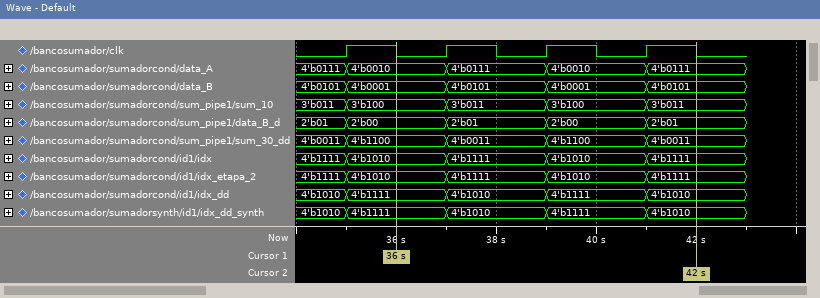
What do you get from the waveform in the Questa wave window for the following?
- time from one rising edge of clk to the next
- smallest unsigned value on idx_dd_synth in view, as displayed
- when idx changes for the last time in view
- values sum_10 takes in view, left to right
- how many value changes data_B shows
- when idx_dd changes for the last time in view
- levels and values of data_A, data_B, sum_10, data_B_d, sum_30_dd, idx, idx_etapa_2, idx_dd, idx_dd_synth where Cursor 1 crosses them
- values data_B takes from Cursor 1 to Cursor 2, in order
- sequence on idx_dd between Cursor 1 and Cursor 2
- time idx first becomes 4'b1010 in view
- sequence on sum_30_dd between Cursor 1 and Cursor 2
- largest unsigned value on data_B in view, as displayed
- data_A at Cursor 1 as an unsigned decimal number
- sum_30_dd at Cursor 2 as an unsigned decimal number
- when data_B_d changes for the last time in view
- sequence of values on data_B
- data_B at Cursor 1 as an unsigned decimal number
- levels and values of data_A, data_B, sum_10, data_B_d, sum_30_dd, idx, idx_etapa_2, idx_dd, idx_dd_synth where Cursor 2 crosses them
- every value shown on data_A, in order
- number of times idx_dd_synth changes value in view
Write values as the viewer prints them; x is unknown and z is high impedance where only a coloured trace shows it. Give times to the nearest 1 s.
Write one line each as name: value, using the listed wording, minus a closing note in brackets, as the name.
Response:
time from one rising edge of clk to the next: 2 s
smallest unsigned value on idx_dd_synth in view, as displayed: 4'b1010
when idx changes for the last time in view: 41 s
values sum_10 takes in view, left to right: 3'b011, 3'b100, 3'b011, 3'b100, 3'b011
how many value changes data_B shows: 4
when idx_dd changes for the last time in view: 41 s
levels and values of data_A, data_B, sum_10, data_B_d, sum_30_dd, idx, idx_etapa_2, idx_dd, idx_dd_synth where Cursor 1 crosses them: data_A=4'b0010, data_B=4'b0001, sum_10=3'b100, data_B_d=2'b00, sum_30_dd=4'b1100, idx=4'b1010, idx_etapa_2=4'b1010, idx_dd=4'b1111, idx_dd_synth=4'b1111
values data_B takes from Cursor 1 to Cursor 2, in order: 4'b0001, 4'b0101, 4'b0001, 4'b0101
sequence on idx_dd between Cursor 1 and Cursor 2: 4'b1111, 4'b1010, 4'b1111, 4'b1010
time idx first becomes 4'b1010 in view: 35 s
sequence on sum_30_dd between Cursor 1 and Cursor 2: 4'b1100, 4'b0011, 4'b1100, 4'b0011
largest unsigned value on data_B in view, as displayed: 4'b0101
data_A at Cursor 1 as an unsigned decimal number: 2
sum_30_dd at Cursor 2 as an unsigned decimal number: 3
when data_B_d changes for the last time in view: 41 s
sequence of values on data_B: 4'b0101, 4'b0001, 4'b0101, 4'b0001, 4'b0101
data_B at Cursor 1 as an unsigned decimal number: 1
levels and values of data_A, data_B, sum_10, data_B_d, sum_30_dd, idx, idx_etapa_2, idx_dd, idx_dd_synth where Cursor 2 crosses them: data_A=4'b0111, data_B=4'b0101, sum_10=3'b011, data_B_d=2'b01, sum_30_dd=4'b0011, idx=4'b1111, idx_etapa_2=4'b1111, idx_dd=4'b1010, idx_dd_synth=4'b1010
every value shown on data_A, in order: 4'b0111, 4'b0010, 4'b0111, 4'b0010, 4'b0111
number of times idx_dd_synth changes value in view: 4
